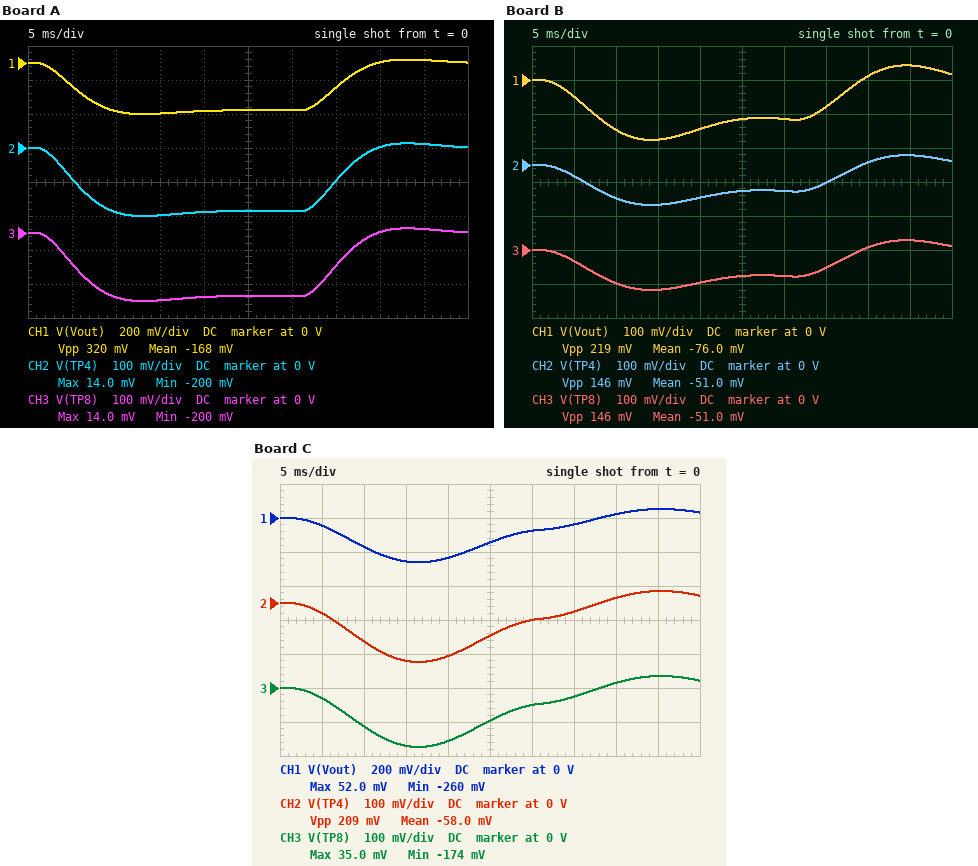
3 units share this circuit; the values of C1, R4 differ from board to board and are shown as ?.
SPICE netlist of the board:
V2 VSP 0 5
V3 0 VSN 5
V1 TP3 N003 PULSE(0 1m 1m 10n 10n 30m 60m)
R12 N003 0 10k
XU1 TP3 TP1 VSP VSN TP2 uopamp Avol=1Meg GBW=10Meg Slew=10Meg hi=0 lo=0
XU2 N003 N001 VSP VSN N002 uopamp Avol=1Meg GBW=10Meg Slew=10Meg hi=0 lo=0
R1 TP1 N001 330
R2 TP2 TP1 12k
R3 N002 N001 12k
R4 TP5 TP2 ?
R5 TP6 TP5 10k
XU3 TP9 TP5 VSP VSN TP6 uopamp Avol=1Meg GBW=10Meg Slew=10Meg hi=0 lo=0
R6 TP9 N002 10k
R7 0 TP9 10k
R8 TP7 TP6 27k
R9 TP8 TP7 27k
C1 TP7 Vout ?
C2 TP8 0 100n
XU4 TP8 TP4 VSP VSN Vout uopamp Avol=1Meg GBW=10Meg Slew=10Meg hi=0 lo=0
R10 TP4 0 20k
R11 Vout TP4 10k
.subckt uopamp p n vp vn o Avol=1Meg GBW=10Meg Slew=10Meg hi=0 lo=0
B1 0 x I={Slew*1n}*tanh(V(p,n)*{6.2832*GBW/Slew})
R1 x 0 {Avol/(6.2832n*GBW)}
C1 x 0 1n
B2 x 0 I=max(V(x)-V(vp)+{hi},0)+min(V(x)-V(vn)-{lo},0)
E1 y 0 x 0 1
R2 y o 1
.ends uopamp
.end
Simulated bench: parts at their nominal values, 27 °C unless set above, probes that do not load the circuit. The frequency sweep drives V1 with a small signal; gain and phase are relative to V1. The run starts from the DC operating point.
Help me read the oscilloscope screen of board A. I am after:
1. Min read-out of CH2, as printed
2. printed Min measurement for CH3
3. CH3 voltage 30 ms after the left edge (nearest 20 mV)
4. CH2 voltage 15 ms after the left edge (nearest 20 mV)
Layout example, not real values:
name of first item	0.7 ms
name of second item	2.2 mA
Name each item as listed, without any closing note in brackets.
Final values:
Min read-out of CH2, as printed	-200 mV
printed Min measurement for CH3	-200 mV
CH3 voltage 30 ms after the left edge	-180 mV
CH2 voltage 15 ms after the left edge	-200 mV
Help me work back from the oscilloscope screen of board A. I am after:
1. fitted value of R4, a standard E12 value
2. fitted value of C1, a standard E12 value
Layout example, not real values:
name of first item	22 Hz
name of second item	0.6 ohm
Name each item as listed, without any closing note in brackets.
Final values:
fitted value of R4, a standard E12 value	3.3 kΩ
fitted value of C1, a standard E12 value	120 nF
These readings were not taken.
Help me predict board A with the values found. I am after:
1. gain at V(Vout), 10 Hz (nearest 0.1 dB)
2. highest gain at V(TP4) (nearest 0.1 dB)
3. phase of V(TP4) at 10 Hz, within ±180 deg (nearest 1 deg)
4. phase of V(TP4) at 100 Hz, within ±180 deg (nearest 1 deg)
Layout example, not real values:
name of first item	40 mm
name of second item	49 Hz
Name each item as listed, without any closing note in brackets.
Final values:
gain at V(Vout), 10 Hz	49.0 dB
highest gain at V(TP4)	45.6 dB
phase of V(TP4) at 10 Hz, within ±180 deg	166 deg
phase of V(TP4) at 100 Hz, within ±180 deg	44 deg
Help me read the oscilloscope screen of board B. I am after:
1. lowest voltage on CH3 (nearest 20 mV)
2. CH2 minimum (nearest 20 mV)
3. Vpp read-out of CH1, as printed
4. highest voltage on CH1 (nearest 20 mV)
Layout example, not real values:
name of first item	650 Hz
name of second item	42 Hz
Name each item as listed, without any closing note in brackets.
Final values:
lowest voltage on CH3	-120 mV
CH2 minimum	-120 mV
Vpp read-out of CH1, as printed	219 mV
highest voltage on CH1	40 mV
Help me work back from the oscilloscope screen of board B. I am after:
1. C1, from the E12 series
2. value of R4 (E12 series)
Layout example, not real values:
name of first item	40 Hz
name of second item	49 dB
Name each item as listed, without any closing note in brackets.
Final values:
C1, from the E12 series	220 nF
value of R4	8.2 kΩ
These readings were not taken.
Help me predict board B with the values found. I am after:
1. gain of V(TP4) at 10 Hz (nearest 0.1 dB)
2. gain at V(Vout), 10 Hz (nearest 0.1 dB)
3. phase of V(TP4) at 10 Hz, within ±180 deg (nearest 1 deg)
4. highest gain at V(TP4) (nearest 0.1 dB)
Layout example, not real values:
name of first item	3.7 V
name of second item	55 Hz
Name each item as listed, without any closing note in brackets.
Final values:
gain of V(TP4) at 10 Hz	39.1 dB
gain at V(Vout), 10 Hz	42.7 dB
phase of V(TP4) at 10 Hz, within ±180 deg	171 deg
highest gain at V(TP4)	43.4 dB
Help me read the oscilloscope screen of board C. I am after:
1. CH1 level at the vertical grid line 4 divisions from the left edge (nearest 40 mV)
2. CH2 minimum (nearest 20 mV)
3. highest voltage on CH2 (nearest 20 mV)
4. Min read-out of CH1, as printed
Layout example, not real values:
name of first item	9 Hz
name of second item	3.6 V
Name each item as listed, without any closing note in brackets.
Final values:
CH1 level at the vertical grid line 4 divisions from the left edge	-240 mV
CH2 minimum	-180 mV
highest voltage on CH2	40 mV
Min read-out of CH1, as printed	-260 mV
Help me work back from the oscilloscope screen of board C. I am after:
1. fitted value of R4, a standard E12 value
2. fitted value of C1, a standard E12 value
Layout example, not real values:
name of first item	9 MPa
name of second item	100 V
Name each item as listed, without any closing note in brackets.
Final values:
fitted value of R4, a standard E12 value	6.8 kΩ
fitted value of C1, a standard E12 value	330 nF
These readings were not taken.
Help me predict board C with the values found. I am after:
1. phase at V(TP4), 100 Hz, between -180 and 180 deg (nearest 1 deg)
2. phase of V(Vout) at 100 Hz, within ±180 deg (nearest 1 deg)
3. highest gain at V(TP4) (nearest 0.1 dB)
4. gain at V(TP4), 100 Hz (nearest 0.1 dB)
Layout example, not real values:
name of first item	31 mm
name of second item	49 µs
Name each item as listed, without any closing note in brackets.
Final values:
phase at V(TP4), 100 Hz, between -180 and 180 deg	4 deg
phase of V(Vout) at 100 Hz, within ±180 deg	4 deg
highest gain at V(TP4)	54.3 dB
gain at V(TP4), 100 Hz	21.4 dB
